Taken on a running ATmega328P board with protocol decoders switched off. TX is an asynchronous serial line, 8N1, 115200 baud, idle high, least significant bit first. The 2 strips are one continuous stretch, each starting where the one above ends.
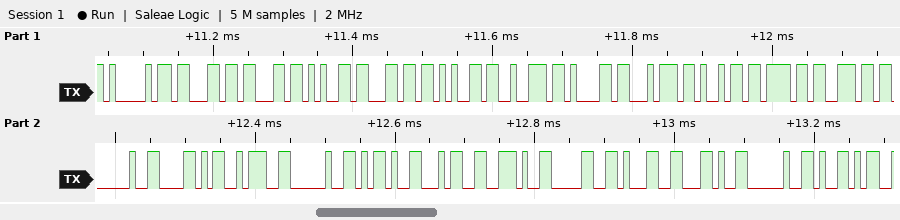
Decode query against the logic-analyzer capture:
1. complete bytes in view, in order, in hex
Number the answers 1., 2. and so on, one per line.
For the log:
1. 41 63 63 65 6C 65 72 61 74 69 6F 6E 20 58 3A 20 2D 34 2E 30 31 2C 20 59
